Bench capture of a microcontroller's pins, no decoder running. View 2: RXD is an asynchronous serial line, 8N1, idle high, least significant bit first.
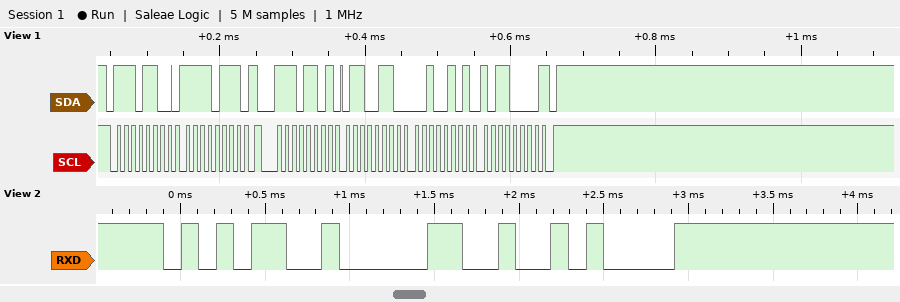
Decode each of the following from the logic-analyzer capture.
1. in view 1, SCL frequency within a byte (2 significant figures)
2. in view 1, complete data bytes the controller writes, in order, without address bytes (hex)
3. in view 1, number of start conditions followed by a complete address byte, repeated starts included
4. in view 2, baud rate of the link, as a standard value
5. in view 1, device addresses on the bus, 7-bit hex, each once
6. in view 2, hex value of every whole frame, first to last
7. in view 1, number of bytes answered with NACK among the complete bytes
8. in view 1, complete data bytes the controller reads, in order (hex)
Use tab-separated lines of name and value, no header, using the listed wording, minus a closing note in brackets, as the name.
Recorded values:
in view 1, SCL frequency within a byte	100 kHz
in view 1, complete data bytes the controller writes, in order, without address bytes	F7
in view 1, number of start conditions followed by a complete address byte, repeated starts included	2
in view 2, baud rate of the link, as a standard value	9600 baud
in view 1, device addresses on the bus, 7-bit hex, each once	0x76
in view 2, hex value of every whole frame, first to last	35 30 0A
in view 1, number of bytes answered with NACK among the complete bytes	1
in view 1, complete data bytes the controller reads, in order	66 25 B0
